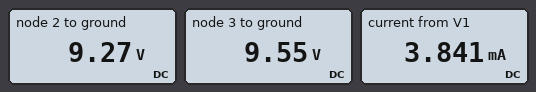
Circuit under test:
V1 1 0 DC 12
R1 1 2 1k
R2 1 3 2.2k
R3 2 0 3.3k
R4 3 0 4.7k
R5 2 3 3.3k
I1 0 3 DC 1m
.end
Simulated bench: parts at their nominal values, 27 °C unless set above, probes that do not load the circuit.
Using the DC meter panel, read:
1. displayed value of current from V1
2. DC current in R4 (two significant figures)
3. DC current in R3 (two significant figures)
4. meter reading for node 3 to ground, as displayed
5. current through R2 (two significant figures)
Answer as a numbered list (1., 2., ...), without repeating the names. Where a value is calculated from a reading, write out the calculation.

1. 3.841 mA
2. (9.55 V) / 4.7 kΩ = 2.0 mA
3. (9.27 V) / 3.3 kΩ = 2.8 mA
4. 9.55 V
5. (12 V - 9.55 V) / 2.2 kΩ = 1.1 mA
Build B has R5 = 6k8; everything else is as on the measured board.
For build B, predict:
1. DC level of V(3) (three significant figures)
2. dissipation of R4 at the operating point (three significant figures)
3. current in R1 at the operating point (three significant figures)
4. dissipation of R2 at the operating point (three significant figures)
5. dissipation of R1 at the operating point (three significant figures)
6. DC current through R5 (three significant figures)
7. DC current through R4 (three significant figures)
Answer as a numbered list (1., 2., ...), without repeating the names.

1. 9.60 V
2. 19.6 mW
3. 2.75 mA
4. 2.63 mW
5. 7.57 mW
6. 51.1 µA
7. 2.04 mA
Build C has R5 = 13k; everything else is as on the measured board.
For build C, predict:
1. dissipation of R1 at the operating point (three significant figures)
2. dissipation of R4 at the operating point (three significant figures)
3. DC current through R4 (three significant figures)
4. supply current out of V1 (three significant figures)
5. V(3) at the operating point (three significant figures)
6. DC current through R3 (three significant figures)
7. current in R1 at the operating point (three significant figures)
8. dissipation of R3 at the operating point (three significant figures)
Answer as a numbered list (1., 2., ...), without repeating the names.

1. 7.66 mW
2. 19.7 mW
3. 2.05 mA
4. 3.85 mA
5. 9.63 V
6. 2.80 mA
7. 2.77 mA
8. 25.8 mW
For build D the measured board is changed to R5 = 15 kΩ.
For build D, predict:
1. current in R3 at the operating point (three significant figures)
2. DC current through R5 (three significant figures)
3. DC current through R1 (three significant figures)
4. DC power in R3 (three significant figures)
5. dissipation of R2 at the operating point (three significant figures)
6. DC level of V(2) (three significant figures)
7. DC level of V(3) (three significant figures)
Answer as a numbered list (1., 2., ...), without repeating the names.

1. 2.80 mA
2. 26.8 µA
3. 2.77 mA
4. 25.8 mW
5. 2.55 mW
6. 9.23 V
7. 9.63 V
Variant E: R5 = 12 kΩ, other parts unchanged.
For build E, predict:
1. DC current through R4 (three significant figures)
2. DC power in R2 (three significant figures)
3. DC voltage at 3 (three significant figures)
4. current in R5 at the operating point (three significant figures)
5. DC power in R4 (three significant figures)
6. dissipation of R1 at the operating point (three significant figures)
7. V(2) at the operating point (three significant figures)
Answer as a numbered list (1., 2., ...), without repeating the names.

1. 2.05 mA
2. 2.57 mW
3. 9.62 V
4. 32.5 µA
5. 19.7 mW
6. 7.65 mW
7. 9.23 V
